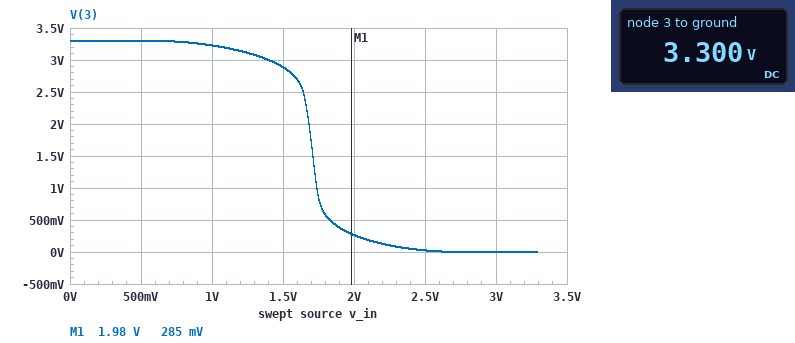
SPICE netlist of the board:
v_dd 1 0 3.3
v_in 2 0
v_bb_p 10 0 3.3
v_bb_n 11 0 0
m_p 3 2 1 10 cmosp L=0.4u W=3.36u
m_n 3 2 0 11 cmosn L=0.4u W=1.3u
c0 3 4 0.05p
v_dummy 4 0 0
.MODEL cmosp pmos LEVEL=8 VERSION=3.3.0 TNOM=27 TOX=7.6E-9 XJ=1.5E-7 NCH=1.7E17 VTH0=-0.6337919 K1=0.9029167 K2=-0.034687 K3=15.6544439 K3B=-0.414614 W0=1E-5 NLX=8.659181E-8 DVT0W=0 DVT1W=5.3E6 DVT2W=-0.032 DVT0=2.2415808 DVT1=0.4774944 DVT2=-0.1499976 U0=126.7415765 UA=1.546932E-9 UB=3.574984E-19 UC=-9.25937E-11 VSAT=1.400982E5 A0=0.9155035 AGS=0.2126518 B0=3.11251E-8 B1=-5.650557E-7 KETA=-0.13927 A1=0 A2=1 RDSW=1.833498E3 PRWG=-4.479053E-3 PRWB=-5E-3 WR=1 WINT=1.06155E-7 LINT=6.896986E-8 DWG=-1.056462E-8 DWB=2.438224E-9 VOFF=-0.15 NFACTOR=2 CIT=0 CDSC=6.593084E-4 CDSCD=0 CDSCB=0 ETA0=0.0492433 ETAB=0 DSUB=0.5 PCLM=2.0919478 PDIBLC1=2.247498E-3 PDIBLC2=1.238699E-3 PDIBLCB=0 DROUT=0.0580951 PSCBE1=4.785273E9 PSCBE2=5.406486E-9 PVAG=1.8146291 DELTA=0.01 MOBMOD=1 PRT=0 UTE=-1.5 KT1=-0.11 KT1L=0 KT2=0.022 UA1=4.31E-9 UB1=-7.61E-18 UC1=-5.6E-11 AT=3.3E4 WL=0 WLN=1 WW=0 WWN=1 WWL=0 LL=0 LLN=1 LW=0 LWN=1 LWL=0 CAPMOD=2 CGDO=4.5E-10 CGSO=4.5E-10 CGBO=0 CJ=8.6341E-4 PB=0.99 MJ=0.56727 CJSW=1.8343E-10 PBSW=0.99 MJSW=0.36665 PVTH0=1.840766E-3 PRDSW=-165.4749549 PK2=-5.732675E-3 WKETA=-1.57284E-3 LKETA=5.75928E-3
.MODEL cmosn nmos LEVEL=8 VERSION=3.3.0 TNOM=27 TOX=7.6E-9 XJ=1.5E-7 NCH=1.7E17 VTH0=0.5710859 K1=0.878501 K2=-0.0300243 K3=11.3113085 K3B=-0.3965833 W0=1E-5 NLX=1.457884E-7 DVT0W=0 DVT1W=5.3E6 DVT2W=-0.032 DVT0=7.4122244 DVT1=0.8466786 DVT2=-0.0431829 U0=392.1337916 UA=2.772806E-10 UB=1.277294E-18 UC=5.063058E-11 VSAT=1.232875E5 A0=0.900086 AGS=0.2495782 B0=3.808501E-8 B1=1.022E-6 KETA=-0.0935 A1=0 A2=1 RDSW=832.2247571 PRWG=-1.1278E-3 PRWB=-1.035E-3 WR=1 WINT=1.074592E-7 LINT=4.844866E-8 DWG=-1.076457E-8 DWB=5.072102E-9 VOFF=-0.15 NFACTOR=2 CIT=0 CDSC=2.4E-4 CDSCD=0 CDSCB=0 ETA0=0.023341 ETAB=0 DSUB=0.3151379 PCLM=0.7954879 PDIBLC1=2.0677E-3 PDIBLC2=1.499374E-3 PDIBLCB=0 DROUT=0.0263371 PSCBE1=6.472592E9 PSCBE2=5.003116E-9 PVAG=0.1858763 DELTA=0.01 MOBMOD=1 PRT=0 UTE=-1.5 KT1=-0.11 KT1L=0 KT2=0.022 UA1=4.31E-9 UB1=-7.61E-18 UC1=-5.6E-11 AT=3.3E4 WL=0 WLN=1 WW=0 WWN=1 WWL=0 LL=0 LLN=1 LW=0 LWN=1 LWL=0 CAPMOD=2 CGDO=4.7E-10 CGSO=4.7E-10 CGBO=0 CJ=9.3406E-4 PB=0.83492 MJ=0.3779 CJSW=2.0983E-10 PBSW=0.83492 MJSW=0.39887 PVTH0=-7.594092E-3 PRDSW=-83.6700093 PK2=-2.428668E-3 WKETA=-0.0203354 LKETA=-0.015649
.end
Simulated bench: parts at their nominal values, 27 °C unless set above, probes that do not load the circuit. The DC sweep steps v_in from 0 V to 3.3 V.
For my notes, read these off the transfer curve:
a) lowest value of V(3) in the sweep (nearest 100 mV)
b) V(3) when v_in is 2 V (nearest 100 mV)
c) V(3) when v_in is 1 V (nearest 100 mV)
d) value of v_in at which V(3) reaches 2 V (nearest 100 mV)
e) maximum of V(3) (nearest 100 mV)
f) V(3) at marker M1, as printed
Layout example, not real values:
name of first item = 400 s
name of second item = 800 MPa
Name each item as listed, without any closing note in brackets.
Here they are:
lowest value of V(3) in the sweep = 0 V
V(3) when v_in is 2 V = 300 mV
V(3) when v_in is 1 V = 3.2 V
value of v_in at which V(3) reaches 2 V = 1.7 V
maximum of V(3) = 3.3 V
V(3) at marker M1, as printed = 285 mV
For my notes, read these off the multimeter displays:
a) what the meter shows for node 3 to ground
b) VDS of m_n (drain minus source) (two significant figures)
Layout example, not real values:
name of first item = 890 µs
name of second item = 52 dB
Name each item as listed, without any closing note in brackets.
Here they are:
what the meter shows for node 3 to ground = 3.300 V
VDS of m_n (drain minus source) = 3.3 V
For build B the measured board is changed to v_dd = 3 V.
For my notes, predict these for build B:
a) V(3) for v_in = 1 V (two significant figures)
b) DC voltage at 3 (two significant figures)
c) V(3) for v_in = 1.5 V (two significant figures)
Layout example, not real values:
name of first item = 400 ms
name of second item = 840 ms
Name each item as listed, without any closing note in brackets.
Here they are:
V(3) for v_in = 1 V = 2.9 V
DC voltage at 3 = 3.0 V
V(3) for v_in = 1.5 V = 1.5 V
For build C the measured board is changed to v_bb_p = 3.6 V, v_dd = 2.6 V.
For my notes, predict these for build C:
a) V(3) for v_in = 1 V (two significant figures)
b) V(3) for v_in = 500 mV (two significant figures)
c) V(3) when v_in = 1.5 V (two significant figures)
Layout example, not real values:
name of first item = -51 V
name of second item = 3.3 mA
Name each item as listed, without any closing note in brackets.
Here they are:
V(3) for v_in = 1 V = 2.5 V
V(3) for v_in = 500 mV = 2.6 V
V(3) when v_in = 1.5 V = 55 mV
